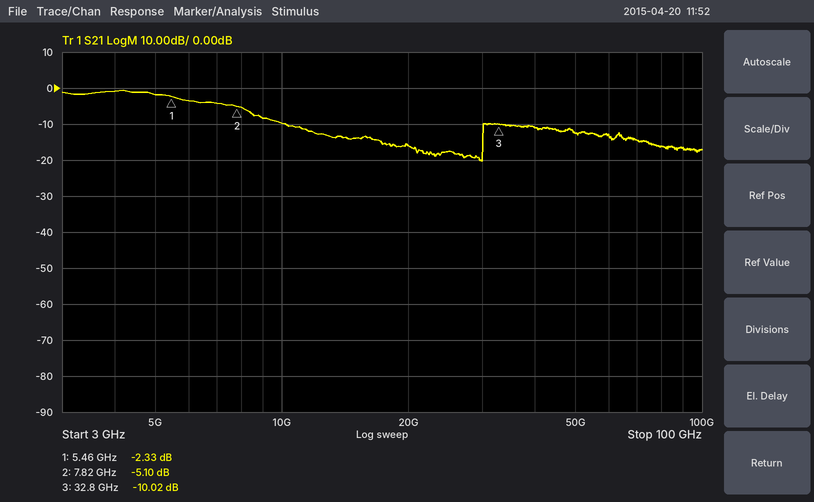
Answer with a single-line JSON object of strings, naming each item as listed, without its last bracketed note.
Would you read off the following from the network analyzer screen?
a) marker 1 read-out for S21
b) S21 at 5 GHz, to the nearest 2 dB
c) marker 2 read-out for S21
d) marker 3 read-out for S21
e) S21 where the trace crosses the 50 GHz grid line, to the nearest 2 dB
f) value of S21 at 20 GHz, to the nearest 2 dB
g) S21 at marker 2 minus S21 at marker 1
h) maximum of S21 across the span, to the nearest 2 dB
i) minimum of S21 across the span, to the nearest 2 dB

{"marker 1 read-out for S21": "-2.33 dB", "S21 at 5 GHz, to the nearest 2 dB": "-2 dB", "marker 2 read-out for S21": "-5.10 dB", "marker 3 read-out for S21": "-10.02 dB", "S21 where the trace crosses the 50 GHz grid line, to the nearest 2 dB": "-12 dB", "value of S21 at 20 GHz, to the nearest 2 dB": "-16 dB", "S21 at marker 2 minus S21 at marker 1": "-2.77 dB", "maximum of S21 across the span, to the nearest 2 dB": "0 dB", "minimum of S21 across the span, to the nearest 2 dB": "-20 dB"}
